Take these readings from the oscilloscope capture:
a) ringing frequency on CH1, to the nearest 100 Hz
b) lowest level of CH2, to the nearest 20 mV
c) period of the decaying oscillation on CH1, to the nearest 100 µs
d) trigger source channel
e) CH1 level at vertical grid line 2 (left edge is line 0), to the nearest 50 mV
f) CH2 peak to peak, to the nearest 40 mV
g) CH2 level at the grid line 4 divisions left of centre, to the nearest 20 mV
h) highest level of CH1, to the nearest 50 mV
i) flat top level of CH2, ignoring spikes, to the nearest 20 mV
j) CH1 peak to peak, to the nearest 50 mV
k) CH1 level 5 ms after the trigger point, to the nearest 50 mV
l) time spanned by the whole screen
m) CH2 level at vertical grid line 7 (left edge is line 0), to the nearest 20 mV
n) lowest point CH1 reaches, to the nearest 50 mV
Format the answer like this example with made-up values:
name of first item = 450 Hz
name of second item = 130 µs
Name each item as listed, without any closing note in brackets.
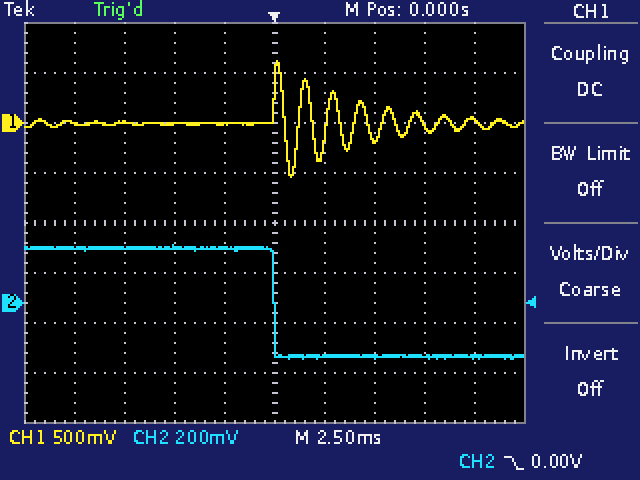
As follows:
ringing frequency on CH1, to the nearest 100 Hz = 700 Hz
lowest level of CH2, to the nearest 20 mV = -220 mV
period of the decaying oscillation on CH1, to the nearest 100 µs = 1.4 ms
trigger source channel = CH2
CH1 level at vertical grid line 2 (left edge is line 0), to the nearest 50 mV = 0 mV
CH2 peak to peak, to the nearest 40 mV = 440 mV
CH2 level at the grid line 4 divisions left of centre, to the nearest 20 mV = 220 mV
highest level of CH1, to the nearest 50 mV = 600 mV
flat top level of CH2, ignoring spikes, to the nearest 20 mV = 220 mV
CH1 peak to peak, to the nearest 50 mV = 1.15 V
CH1 level 5 ms after the trigger point, to the nearest 50 mV = -150 mV
time spanned by the whole screen = 25 ms
CH2 level at vertical grid line 7 (left edge is line 0), to the nearest 20 mV = -220 mV
lowest point CH1 reaches, to the nearest 50 mV = -550 mV
